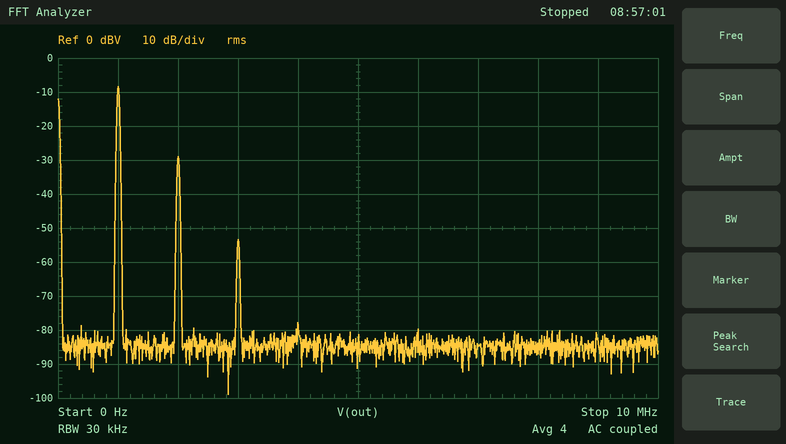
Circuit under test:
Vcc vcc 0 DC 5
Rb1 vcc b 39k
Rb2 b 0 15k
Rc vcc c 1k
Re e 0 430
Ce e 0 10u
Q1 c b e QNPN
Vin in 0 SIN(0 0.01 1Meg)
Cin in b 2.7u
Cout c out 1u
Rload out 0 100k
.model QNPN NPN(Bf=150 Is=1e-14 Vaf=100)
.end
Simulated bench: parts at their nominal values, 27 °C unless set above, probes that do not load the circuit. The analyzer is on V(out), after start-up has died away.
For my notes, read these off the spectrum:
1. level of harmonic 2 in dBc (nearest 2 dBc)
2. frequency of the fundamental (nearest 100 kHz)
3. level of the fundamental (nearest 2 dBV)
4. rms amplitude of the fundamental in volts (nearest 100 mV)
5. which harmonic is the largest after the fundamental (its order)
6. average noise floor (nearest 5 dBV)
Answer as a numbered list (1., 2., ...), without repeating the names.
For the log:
1. -20 dBc
2. 1.0 MHz
3. -8 dBV
4. 400 mV
5. 2
6. -85 dBV
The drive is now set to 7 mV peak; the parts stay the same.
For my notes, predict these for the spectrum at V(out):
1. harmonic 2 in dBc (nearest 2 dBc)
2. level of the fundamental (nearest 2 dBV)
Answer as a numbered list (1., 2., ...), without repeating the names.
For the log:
1. -24 dBc
2. -12 dBV
